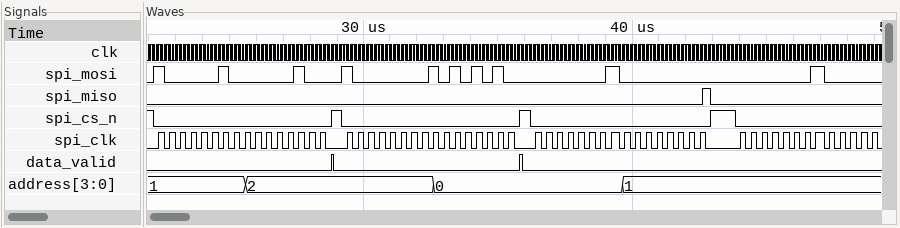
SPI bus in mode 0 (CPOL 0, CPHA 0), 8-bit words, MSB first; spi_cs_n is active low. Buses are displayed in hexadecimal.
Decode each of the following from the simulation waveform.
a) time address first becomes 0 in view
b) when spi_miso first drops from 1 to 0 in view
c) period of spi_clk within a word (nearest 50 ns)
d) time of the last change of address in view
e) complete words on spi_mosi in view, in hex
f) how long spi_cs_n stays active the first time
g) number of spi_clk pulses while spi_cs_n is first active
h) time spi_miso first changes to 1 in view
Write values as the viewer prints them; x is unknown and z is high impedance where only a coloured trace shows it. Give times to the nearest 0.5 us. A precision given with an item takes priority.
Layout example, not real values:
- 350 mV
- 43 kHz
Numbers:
- 32.5 us
- 43 us
- 400 ns
- 39.5 us
- 82, 04, 80, AA, 01, 00, 01
- 6.5 us
- 16
- 42.5 us
